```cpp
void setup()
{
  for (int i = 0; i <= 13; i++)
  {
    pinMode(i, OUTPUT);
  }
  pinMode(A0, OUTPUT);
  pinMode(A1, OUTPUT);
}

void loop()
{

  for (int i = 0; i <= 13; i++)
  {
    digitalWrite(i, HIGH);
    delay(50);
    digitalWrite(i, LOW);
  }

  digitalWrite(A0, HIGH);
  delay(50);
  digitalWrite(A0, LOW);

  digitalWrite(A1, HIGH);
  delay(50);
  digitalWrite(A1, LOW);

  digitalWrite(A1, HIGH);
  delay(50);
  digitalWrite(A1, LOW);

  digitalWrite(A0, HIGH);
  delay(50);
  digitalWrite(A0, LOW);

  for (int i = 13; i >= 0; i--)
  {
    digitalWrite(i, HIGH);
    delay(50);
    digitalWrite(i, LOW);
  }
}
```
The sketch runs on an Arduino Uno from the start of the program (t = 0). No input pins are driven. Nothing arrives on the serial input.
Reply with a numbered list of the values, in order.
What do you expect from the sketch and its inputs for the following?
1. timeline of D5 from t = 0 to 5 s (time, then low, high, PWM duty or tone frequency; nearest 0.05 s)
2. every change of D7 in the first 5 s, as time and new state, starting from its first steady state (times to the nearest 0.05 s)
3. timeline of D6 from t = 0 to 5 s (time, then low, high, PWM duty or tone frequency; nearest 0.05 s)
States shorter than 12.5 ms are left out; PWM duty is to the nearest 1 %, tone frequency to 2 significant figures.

1. 0 s low; 0.25 s high; 0.3 s low; 1.3 s high; 1.35 s low; 1.85 s high; 1.9 s low; 2.9 s high; 2.95 s low; 3.45 s high; 3.5 s low; 4.5 s high; 4.55 s low
2. 0 s low; 0.35 s high; 0.4 s low; 1.2 s high; 1.25 s low; 1.95 s high; 2 s low; 2.8 s high; 2.85 s low; 3.55 s high; 3.6 s low; 4.4 s high; 4.45 s low
3. 0 s low; 0.3 s high; 0.35 s low; 1.25 s high; 1.3 s low; 1.9 s high; 1.95 s low; 2.85 s high; 2.9 s low; 3.5 s high; 3.55 s low; 4.45 s high; 4.5 s low
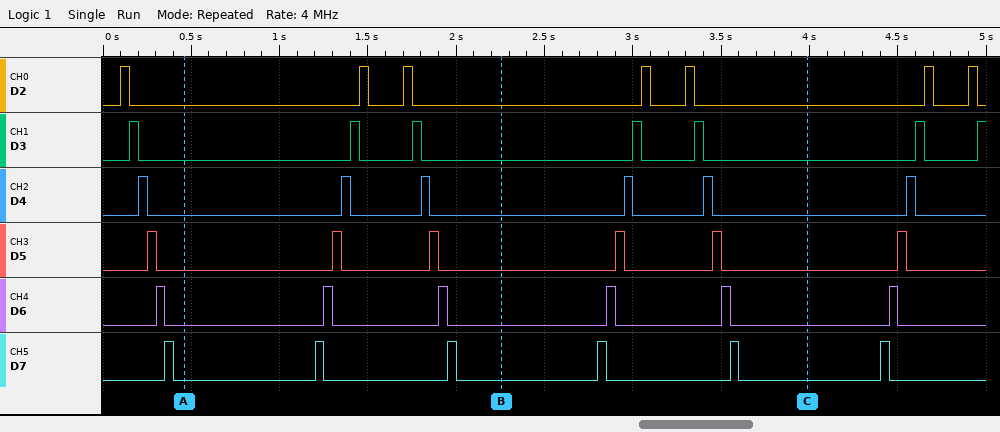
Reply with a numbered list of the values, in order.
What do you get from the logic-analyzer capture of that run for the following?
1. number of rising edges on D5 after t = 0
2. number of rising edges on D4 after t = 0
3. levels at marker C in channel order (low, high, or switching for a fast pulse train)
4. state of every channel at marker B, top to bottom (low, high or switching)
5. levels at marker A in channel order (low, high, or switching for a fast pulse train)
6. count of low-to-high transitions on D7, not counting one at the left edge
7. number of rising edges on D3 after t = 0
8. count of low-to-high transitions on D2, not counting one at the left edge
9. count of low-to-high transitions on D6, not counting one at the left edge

1. 6
2. 6
3. D2 low, D3 low, D4 low, D5 low, D6 low, D7 low
4. D2 low, D3 low, D4 low, D5 low, D6 low, D7 low
5. D2 low, D3 low, D4 low, D5 low, D6 low, D7 low
6. 6
7. 7
8. 7
9. 6
